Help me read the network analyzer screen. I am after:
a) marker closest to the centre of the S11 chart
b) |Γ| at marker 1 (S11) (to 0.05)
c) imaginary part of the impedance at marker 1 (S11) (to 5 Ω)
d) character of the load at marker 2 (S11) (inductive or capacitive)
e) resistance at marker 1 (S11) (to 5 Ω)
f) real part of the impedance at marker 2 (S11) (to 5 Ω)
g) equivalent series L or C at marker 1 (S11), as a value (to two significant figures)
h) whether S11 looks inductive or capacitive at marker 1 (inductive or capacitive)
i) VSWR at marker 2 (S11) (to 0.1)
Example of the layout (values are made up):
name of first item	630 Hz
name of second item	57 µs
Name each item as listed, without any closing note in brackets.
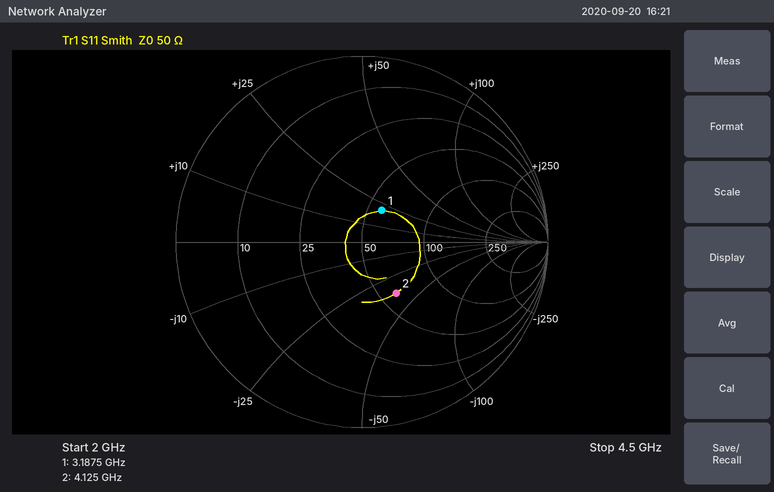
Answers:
marker closest to the centre of the S11 chart	marker 1
|Γ| at marker 1 (S11)	0.20
imaginary part of the impedance at marker 1 (S11)	+20 Ω
character of the load at marker 2 (S11)	capacitive
resistance at marker 1 (S11)	60 Ω
real part of the impedance at marker 2 (S11)	60 Ω
equivalent series L or C at marker 1 (S11), as a value	1.0 nH
whether S11 looks inductive or capacitive at marker 1	inductive
VSWR at marker 2 (S11)	2.0
